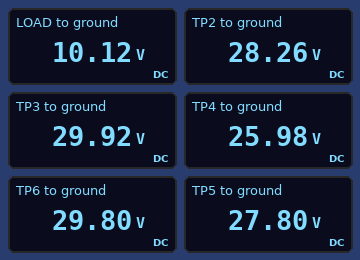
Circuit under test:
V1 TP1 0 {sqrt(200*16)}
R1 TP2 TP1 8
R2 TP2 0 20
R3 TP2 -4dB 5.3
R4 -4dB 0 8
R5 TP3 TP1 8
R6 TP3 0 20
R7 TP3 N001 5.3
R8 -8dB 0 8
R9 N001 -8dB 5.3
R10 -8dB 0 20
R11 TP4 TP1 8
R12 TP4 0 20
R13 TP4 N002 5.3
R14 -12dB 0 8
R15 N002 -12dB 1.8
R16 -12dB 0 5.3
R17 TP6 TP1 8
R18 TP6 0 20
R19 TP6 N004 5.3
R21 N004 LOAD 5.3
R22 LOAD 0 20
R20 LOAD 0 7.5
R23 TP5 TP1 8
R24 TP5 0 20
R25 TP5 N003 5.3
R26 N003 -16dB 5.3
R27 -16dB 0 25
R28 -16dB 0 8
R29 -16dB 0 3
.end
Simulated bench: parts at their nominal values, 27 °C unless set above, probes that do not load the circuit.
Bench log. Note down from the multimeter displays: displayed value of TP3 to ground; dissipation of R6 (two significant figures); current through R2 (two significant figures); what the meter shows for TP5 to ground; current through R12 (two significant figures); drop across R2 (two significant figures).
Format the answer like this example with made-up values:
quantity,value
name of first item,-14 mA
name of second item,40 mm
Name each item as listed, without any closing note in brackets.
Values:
quantity,value
displayed value of TP3 to ground,29.92 V
dissipation of R6,45 W
current through R2,1.4 A
what the meter shows for TP5 to ground,27.80 V
current through R12,1.3 A
drop across R2,28 V
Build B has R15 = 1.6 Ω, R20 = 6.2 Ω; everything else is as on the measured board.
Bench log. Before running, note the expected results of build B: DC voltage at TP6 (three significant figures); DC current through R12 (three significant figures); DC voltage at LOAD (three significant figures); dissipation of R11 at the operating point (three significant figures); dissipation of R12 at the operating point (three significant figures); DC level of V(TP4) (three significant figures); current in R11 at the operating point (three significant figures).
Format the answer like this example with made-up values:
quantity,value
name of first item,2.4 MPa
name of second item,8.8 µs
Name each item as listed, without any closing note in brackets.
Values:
quantity,value
DC voltage at TP6,29.4 V
DC current through R12,1.29 A
DC voltage at LOAD,9.09 V
dissipation of R11 at the operating point,118 W
dissipation of R12 at the operating point,33.3 W
DC level of V(TP4),25.8 V
current in R11 at the operating point,3.85 A
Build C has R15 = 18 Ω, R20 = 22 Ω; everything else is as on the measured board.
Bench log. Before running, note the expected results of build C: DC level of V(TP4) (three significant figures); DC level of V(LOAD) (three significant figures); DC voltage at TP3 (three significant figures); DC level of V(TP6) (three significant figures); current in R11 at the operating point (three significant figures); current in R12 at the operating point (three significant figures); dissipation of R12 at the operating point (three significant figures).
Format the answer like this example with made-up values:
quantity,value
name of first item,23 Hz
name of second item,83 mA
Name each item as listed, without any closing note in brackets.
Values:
quantity,value
DC level of V(TP4),33.2 V
DC level of V(LOAD),15.8 V
DC voltage at TP3,29.9 V
DC level of V(TP6),31.8 V
current in R11 at the operating point,2.92 A
current in R12 at the operating point,1.66 A
dissipation of R12 at the operating point,55.2 W
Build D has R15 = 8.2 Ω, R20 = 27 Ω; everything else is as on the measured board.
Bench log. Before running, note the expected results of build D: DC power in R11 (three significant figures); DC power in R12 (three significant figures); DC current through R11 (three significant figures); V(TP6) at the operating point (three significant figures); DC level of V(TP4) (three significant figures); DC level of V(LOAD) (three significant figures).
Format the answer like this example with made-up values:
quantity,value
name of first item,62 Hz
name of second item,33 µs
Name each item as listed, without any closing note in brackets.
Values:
quantity,value
DC power in R11,87.6 W
DC power in R12,45.3 W
DC current through R11,3.31 A
V(TP6) at the operating point,32.1 V
DC level of V(TP4),30.1 V
DC level of V(LOAD),16.7 V
